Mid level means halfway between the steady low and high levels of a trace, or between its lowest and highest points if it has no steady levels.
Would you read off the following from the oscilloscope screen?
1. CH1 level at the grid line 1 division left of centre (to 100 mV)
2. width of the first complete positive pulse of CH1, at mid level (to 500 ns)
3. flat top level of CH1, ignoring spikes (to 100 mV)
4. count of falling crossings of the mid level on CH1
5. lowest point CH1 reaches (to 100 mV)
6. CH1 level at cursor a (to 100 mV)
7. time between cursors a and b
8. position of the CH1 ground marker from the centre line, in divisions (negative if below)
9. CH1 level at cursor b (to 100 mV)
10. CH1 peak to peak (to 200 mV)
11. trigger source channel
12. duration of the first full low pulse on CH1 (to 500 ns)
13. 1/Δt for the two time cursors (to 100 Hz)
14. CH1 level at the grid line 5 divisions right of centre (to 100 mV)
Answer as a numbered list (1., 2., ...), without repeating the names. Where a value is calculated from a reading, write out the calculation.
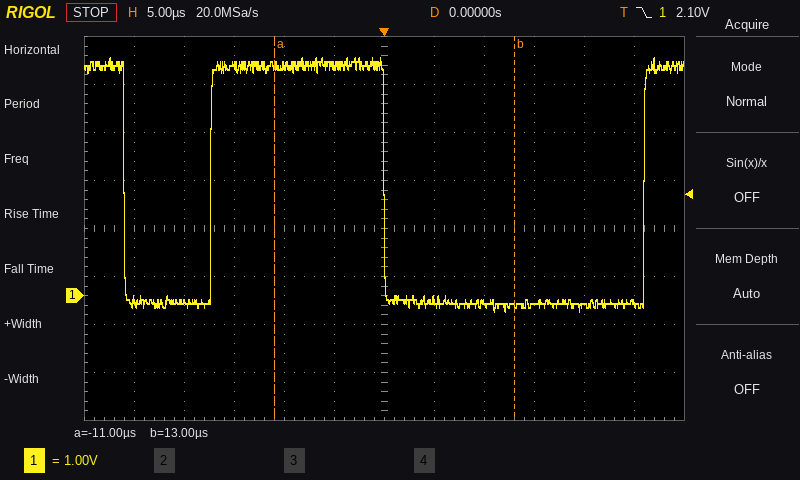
1. 4.8 V
2. 17.5 µs
3. 4.8 V
4. 2
5. -300 mV
6. 4.8 V
7. 13 µs − (-11 µs) = 24.0 µs
8. -1.4 div
9. -200 mV
10. 5.2 V
11. CH1
12. 8.5 µs
13. 1 / 24.0 µs ≈ 41.7 kHz
14. -200 mV
